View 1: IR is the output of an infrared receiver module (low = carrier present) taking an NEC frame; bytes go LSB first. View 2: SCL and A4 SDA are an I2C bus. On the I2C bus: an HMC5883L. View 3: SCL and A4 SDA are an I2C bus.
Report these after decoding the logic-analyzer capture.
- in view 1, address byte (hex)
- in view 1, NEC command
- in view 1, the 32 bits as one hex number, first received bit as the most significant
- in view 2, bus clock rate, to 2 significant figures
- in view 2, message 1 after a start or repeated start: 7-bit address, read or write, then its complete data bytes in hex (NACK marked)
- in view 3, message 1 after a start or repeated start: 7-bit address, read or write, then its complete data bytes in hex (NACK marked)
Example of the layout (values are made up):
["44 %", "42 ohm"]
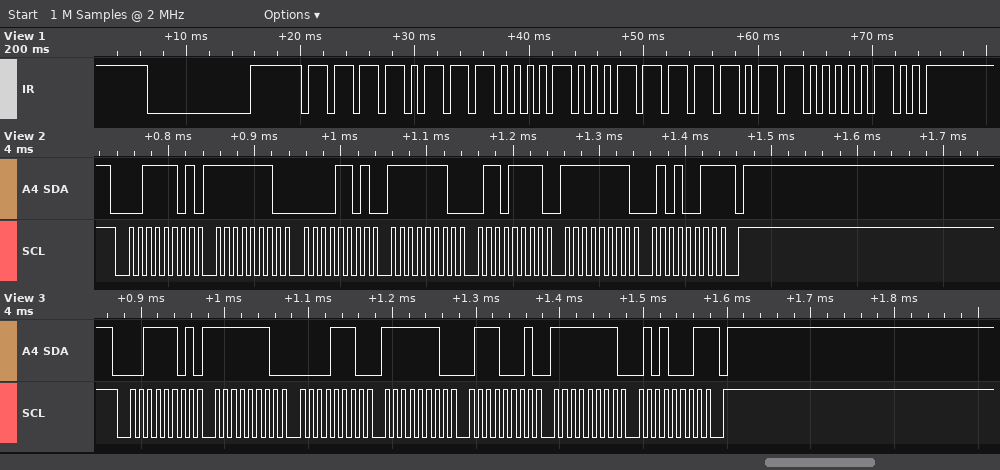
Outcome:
["0xEF", "0xDF", "0xF708FB04", "100 kHz", "0x1E read: FE 0D FE 6F FF 53 NACK", "0x1E read: FE 0E FE 71 FF 51 NACK"]
